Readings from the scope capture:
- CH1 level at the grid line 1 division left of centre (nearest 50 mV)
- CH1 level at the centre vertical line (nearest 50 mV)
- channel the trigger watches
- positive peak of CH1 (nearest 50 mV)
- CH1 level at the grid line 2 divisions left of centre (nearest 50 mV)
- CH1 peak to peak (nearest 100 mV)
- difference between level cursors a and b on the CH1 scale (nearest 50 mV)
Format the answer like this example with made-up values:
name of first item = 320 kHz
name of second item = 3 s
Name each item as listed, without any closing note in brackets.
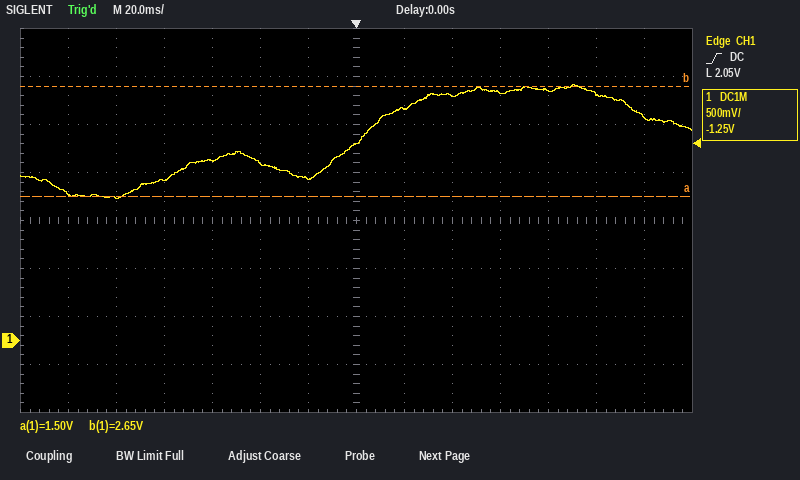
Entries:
CH1 level at the grid line 1 division left of centre = 1.70 V
CH1 level at the centre vertical line = 2.05 V
channel the trigger watches = CH1
positive peak of CH1 = 2.65 V
CH1 level at the grid line 2 divisions left of centre = 1.85 V
CH1 peak to peak = 1.20 V
difference between level cursors a and b on the CH1 scale = 1.15 V
